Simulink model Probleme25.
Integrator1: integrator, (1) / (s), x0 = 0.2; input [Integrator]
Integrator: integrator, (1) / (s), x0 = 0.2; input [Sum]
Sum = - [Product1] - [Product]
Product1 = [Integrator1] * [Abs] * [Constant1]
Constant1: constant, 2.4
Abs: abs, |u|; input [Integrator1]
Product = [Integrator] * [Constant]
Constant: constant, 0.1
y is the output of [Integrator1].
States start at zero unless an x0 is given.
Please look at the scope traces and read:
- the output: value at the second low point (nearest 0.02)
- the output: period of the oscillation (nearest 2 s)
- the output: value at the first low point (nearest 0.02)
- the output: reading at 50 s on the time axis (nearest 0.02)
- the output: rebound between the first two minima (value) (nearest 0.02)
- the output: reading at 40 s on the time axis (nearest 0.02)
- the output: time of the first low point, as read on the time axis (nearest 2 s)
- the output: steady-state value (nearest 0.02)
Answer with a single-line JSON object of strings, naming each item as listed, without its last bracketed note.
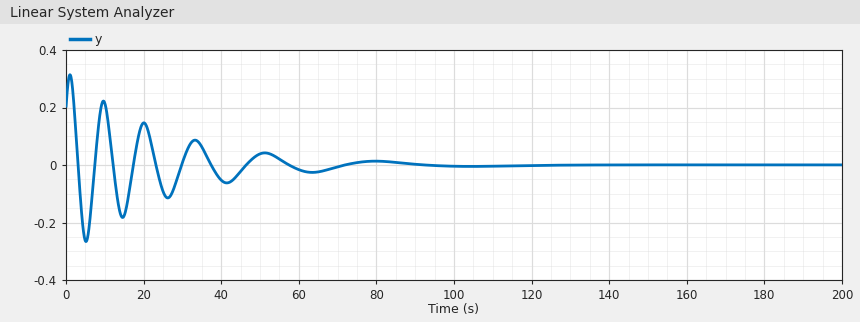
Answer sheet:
{"the output: value at the second low point": "-0.18", "the output: period of the oscillation": "10 s", "the output: value at the first low point": "-0.26", "the output: reading at 50 s on the time axis": "0.04", "the output: rebound between the first two minima (value)": "0.22", "the output: reading at 40 s on the time axis": "-0.06", "the output: time of the first low point, as read on the time axis": "6 s", "the output: steady-state value": "0.00"}
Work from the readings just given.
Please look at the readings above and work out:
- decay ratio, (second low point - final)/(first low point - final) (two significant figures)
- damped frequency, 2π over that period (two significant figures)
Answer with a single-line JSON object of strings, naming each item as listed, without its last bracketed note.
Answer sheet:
{"decay ratio, (second low point - final)/(first low point - final)": "0.69", "damped frequency, 2π over that period": "0.63 rad/s"}
